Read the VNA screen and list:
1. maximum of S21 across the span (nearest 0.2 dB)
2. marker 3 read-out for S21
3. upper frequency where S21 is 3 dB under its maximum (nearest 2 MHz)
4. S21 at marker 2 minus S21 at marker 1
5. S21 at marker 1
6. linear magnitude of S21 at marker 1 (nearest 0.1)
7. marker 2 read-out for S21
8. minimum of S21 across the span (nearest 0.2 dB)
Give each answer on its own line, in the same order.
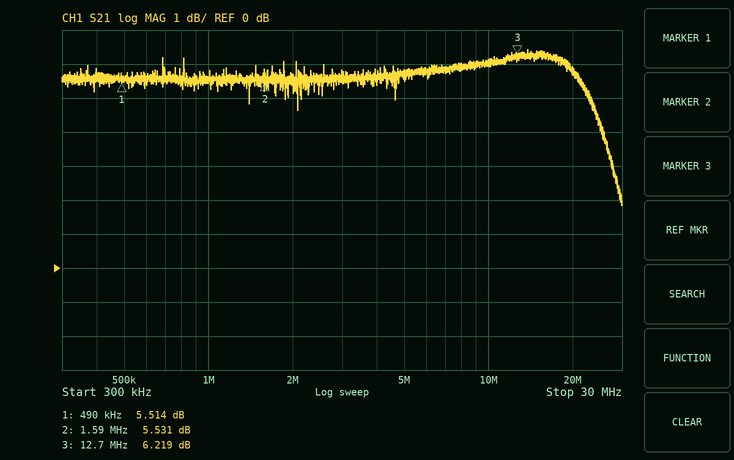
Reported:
6.4 dB
6.219 dB
26 MHz
0.017 dB
5.514 dB
1.9
5.531 dB
1.8 dB
